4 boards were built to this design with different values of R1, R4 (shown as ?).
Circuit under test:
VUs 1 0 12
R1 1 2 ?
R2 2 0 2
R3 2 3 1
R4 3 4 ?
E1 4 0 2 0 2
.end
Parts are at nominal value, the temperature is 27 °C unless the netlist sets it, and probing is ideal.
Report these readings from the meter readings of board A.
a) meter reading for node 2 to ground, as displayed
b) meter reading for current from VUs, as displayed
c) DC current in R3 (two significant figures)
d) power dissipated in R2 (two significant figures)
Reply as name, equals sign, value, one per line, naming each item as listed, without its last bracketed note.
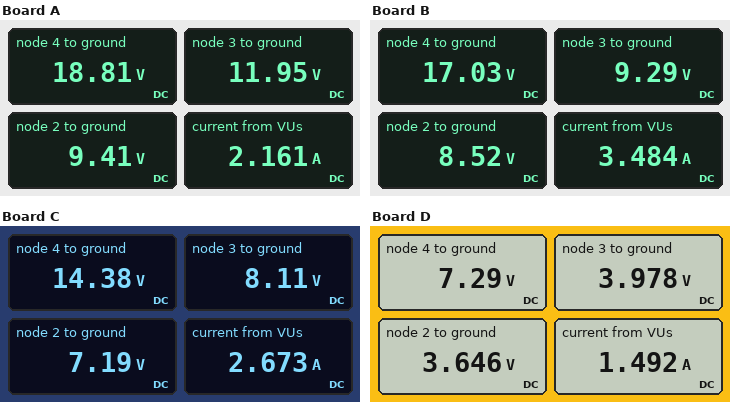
meter reading for node 2 to ground, as displayed = 9.41 V
meter reading for current from VUs, as displayed = 2.161 A
DC current in R3 = 2.5 A
power dissipated in R2 = 44 W
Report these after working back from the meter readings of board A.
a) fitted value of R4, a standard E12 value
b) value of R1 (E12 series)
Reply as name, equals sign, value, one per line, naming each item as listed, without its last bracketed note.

fitted value of R4, a standard E12 value = 2.7 Ω
value of R1 = 1.2 Ω
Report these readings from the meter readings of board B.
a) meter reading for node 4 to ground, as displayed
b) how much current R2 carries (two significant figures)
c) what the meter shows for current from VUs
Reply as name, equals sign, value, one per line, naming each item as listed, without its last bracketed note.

meter reading for node 4 to ground, as displayed = 17.03 V
how much current R2 carries = 4.3 A
what the meter shows for current from VUs = 3.484 A
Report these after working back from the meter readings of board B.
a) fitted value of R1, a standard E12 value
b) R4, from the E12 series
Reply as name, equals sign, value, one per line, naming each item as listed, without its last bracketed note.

fitted value of R1, a standard E12 value = 1 Ω
R4, from the E12 series = 10 Ω
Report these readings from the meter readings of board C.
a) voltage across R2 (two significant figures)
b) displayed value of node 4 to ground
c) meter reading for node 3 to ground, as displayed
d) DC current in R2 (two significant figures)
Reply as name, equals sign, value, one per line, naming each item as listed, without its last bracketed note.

voltage across R2 = 7.2 V
displayed value of node 4 to ground = 14.38 V
meter reading for node 3 to ground, as displayed = 8.11 V
DC current in R2 = 3.6 A
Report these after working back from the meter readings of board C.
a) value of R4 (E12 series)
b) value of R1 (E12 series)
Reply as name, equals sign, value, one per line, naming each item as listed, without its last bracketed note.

value of R4 = 6.8 Ω
value of R1 = 1.8 Ω
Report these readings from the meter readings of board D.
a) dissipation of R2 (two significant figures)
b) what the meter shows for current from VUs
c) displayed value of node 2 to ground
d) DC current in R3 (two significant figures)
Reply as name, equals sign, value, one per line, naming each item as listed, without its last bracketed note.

dissipation of R2 = 6.6 W
what the meter shows for current from VUs = 1.492 A
displayed value of node 2 to ground = 3.646 V
DC current in R3 = 330 mA
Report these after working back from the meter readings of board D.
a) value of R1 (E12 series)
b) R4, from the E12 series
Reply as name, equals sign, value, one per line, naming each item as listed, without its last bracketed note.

value of R1 = 5.6 Ω
R4, from the E12 series = 10 Ω
